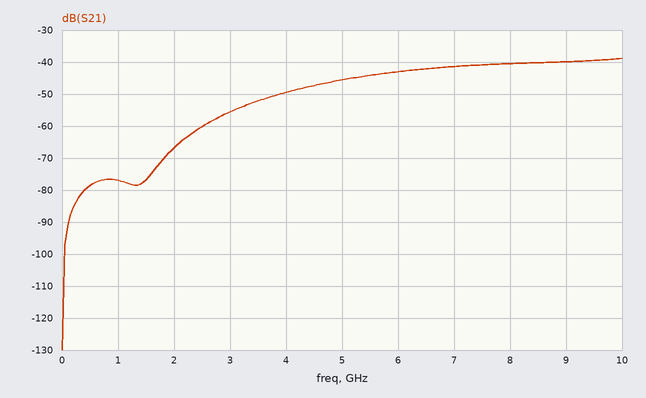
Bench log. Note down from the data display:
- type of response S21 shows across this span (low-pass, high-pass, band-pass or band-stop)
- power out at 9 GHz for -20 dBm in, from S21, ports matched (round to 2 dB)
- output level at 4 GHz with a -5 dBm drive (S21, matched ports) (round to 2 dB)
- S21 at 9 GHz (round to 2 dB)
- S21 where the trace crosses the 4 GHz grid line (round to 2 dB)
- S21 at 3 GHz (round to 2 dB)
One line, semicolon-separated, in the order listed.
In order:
high-pass; -60 dBm; -54 dBm; -40 dB; -50 dB; -56 dB
